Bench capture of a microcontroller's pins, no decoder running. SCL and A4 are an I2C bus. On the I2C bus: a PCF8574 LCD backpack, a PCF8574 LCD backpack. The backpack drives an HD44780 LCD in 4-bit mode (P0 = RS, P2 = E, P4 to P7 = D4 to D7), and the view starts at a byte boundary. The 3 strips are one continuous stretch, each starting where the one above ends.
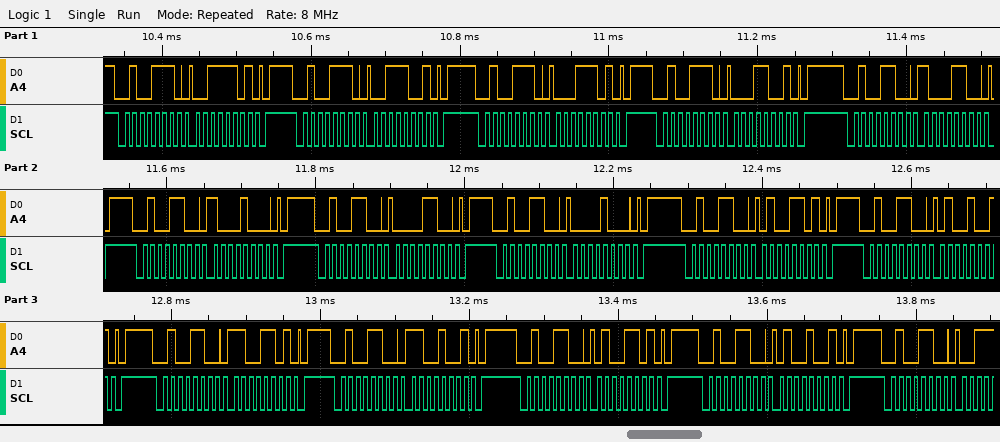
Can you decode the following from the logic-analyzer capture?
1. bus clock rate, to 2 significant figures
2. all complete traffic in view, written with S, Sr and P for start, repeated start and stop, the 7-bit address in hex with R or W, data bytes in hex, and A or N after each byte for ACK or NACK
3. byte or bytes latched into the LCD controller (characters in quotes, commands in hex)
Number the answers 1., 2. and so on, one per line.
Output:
1. 100 kHz
2. S 27W A 3D A P S 27W A 39 A P S 27W A 1D A P S 27W A 19 A P S 26W A 8C A P S 26W A 88 A P S 26W A 0C A P S 26W A 08 A P S 26W A 4D A P S 26W A 49 A P S 26W A CD A P S 26W A C9 A P S 26W A 4D A P S 26W A 49 A P S 26W A
3. '1' 0x80 'L'
